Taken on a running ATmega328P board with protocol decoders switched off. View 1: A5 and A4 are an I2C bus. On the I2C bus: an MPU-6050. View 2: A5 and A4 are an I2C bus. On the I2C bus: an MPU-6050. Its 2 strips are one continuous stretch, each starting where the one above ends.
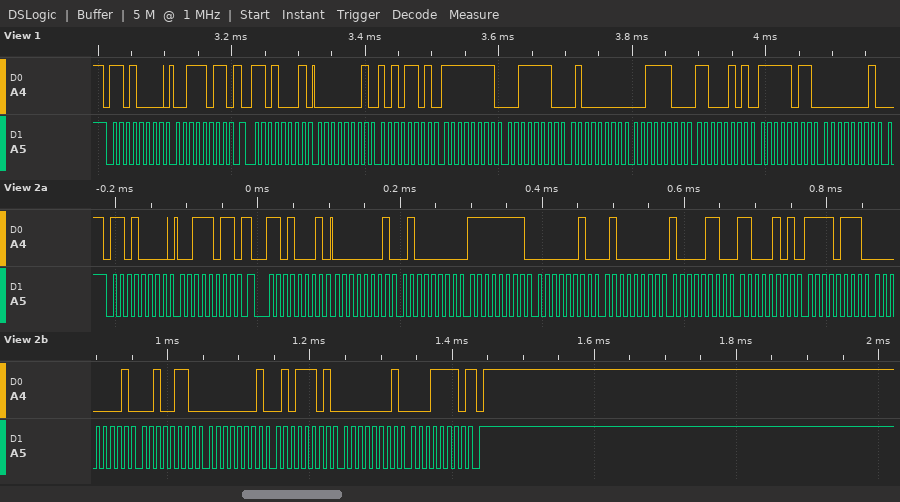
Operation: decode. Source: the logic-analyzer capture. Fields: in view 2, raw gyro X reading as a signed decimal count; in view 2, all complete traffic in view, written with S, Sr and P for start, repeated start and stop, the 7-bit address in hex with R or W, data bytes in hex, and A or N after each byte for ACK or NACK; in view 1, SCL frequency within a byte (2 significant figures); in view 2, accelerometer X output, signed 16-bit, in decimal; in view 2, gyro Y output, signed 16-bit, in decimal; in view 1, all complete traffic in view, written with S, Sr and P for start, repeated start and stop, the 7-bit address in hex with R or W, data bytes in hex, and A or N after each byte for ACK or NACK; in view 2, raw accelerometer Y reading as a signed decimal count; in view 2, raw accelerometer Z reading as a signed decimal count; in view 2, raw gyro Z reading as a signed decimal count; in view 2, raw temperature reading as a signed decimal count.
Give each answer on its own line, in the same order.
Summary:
294
S 68W A 3B A Sr 68R A 01 A 40 A FF A 02 A 40 A 86 A C5 A F7 A 01 A 26 A 01 A 5D A 01 A 1E N P
100 kHz
320
349
S 68W A 3B A Sr 68R A 01 A AD A FF A 3E A 40 A 3C A C5 A FB A 01 A
-254
16518
286
-14857
